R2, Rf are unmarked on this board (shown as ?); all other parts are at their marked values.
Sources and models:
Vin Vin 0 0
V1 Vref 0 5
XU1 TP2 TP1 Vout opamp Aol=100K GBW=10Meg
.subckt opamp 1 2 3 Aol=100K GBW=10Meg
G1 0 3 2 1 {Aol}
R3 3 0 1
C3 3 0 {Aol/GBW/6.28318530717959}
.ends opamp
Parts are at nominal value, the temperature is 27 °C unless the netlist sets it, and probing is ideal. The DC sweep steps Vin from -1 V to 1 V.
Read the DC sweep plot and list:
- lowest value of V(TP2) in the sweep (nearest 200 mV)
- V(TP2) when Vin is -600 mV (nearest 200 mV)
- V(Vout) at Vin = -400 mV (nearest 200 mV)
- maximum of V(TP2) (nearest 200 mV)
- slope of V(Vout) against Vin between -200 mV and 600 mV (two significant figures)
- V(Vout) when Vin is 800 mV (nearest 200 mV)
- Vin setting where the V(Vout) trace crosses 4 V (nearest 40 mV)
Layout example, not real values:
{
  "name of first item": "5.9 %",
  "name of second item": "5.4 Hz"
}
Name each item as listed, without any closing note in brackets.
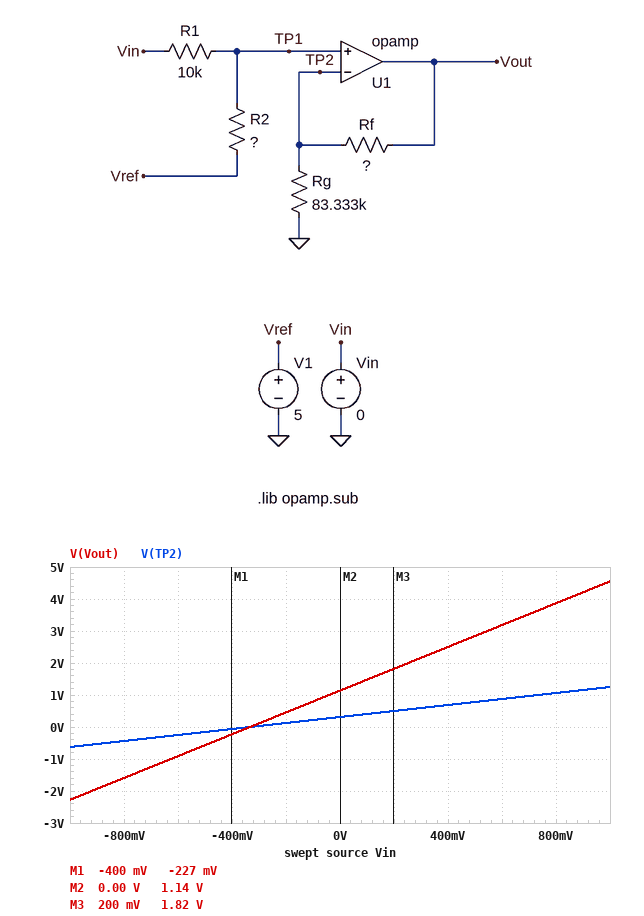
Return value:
{
  "lowest value of V(TP2) in the sweep": "-600 mV",
  "V(TP2) when Vin is -600 mV": "-200 mV",
  "V(Vout) at Vin = -400 mV": "-200 mV",
  "maximum of V(TP2)": "1.2 V",
  "slope of V(Vout) against Vin between -200 mV and 600 mV": "3.4 V/V",
  "V(Vout) when Vin is 800 mV": "3.8 V",
  "Vin setting where the V(Vout) trace crosses 4 V": "840 mV"
}
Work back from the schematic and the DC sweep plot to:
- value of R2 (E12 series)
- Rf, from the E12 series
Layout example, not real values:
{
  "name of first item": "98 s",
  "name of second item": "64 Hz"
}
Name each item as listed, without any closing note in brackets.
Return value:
{
  "value of R2": "150 kΩ",
  "Rf, from the E12 series": "220 kΩ"
}
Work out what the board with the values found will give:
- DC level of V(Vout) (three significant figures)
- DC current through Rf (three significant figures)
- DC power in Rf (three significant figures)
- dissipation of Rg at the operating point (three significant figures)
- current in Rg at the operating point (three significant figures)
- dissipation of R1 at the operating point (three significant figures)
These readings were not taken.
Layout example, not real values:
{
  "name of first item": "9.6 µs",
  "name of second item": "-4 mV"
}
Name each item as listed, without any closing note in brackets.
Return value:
{
  "DC level of V(Vout)": "1.14 V",
  "DC current through Rf": "3.75 µA",
  "DC power in Rf": "3.09 µW",
  "dissipation of Rg at the operating point": "1.17 µW",
  "current in Rg at the operating point": "3.75 µA",
  "dissipation of R1 at the operating point": "9.77 µW"
}
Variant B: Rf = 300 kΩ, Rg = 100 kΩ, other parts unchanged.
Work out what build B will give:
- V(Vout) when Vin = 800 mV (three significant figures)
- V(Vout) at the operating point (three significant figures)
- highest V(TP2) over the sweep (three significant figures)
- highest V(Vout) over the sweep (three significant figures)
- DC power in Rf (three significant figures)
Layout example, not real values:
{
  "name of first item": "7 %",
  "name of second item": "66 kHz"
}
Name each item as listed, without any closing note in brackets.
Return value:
{
  "V(Vout) when Vin = 800 mV": "4.25 V",
  "V(Vout) at the operating point": "1.25 V",
  "highest V(TP2) over the sweep": "1.25 V",
  "highest V(Vout) over the sweep": "5.00 V",
  "DC power in Rf": "2.93 µW"
}
